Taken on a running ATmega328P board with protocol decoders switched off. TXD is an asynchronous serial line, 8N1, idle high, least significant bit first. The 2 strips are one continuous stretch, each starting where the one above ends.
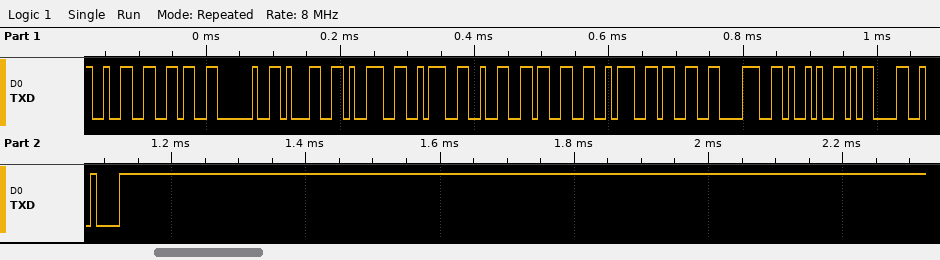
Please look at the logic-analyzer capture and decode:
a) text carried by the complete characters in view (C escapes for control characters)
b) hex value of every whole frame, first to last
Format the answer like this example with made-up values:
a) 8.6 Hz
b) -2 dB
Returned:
a) "26 19:23:38)\r\n"
b) 0x32 0x36 0x20 0x31 0x39 0x3A 0x32 0x33 0x3A 0x33 0x38 0x29 0x0D 0x0A
